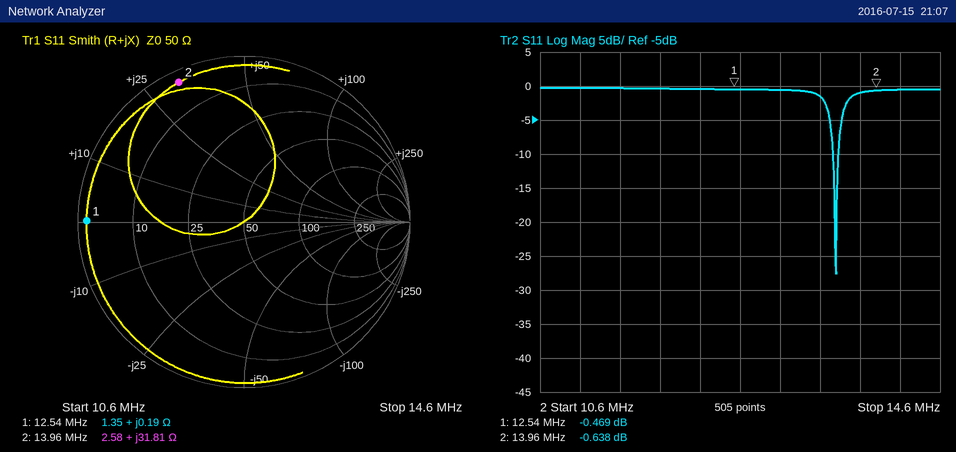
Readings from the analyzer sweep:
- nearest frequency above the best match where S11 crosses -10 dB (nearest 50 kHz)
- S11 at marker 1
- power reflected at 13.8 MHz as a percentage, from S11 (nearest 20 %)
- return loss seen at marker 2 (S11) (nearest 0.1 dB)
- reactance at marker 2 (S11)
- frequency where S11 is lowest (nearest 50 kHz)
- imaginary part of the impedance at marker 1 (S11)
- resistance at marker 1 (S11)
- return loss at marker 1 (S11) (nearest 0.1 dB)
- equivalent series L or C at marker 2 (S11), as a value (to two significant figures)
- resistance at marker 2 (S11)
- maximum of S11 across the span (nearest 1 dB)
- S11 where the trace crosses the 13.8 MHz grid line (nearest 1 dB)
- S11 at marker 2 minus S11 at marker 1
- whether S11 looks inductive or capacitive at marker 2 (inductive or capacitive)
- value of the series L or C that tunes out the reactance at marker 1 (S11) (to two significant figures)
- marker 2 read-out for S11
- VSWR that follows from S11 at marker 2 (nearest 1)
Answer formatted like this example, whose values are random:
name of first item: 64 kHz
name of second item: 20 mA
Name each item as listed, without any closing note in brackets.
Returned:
nearest frequency above the best match where S11 crosses -10 dB: 13.60 MHz
S11 at marker 1: -0.469 dB
power reflected at 13.8 MHz as a percentage, from S11: 80 %
return loss seen at marker 2 (S11): 0.6 dB
reactance at marker 2: +31.81 Ω
frequency where S11 is lowest: 13.55 MHz
imaginary part of the impedance at marker 1: +0.19 Ω
resistance at marker 1: 1.35 Ω
return loss at marker 1 (S11): 0.5 dB
equivalent series L or C at marker 2 (S11), as a value: 360 nH
resistance at marker 2: 2.58 Ω
maximum of S11 across the span: 0 dB
S11 where the trace crosses the 13.8 MHz grid line: -1 dB
S11 at marker 2 minus S11 at marker 1: -0.169 dB
whether S11 looks inductive or capacitive at marker 2: inductive
value of the series L or C that tunes out the reactance at marker 1 (S11): 67 nF
marker 2 read-out for S11: -0.638 dB
VSWR that follows from S11 at marker 2: 27
